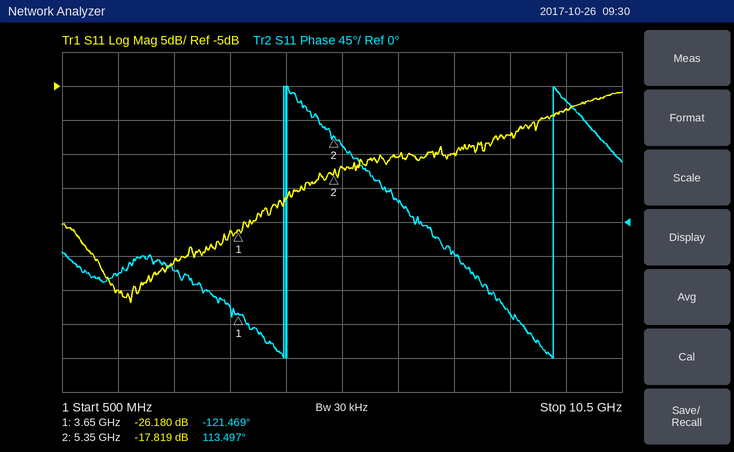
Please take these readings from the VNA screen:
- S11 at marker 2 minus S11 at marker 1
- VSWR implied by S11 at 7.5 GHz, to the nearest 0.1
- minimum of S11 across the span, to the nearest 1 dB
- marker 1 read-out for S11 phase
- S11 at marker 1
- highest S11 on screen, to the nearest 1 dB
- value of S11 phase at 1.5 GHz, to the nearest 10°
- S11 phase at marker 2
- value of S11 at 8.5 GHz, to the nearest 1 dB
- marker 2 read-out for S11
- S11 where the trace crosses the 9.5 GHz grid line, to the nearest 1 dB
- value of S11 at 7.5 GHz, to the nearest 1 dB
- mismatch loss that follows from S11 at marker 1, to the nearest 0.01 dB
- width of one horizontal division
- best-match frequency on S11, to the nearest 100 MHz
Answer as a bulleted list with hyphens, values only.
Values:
- 8.361 dB
- 1.4
- -37 dB
- -121.469°
- -26.180 dB
- -6 dB
- -70°
- 113.497°
- -12 dB
- -17.819 dB
- -8 dB
- -15 dB
- 0.01 dB
- 1 GHz
- 1.7 GHz
